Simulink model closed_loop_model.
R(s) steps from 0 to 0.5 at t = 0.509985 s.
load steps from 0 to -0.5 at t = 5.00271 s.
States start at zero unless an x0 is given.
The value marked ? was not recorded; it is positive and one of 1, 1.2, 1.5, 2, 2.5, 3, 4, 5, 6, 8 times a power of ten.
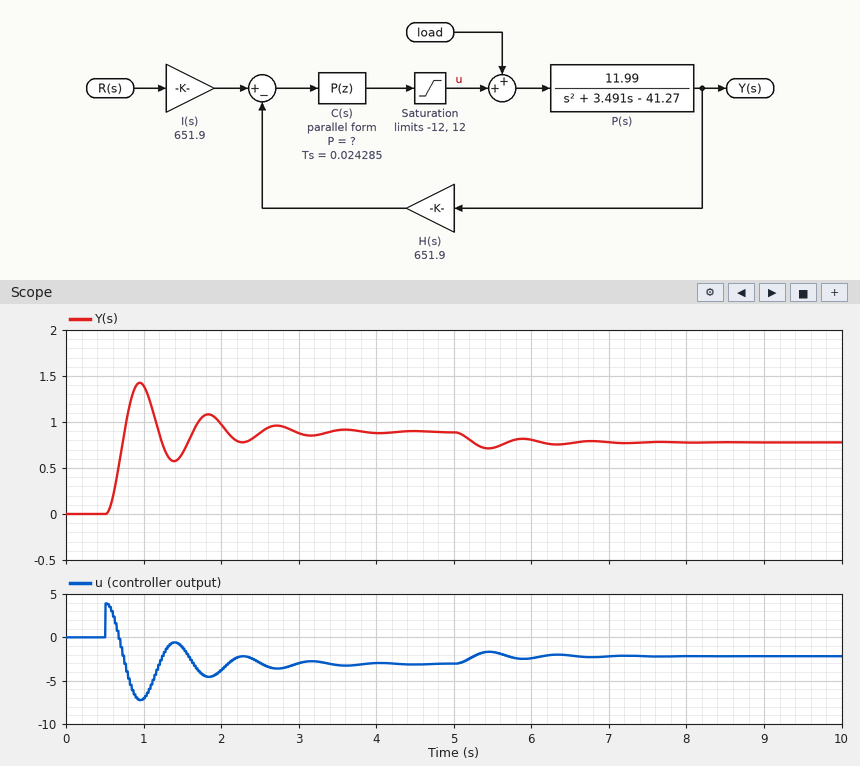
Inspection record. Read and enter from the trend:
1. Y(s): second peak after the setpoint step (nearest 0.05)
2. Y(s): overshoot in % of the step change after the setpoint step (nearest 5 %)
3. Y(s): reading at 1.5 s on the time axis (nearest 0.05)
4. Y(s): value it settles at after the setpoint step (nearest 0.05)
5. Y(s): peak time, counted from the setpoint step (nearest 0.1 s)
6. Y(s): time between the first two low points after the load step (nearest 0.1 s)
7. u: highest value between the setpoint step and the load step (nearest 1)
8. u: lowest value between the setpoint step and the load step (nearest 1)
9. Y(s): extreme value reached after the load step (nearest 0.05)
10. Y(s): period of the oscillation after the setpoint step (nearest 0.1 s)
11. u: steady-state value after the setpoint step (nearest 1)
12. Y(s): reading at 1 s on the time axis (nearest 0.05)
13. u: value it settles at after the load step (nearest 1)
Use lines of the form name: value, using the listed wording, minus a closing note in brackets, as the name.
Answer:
Y(s): second peak after the setpoint step: 1.10
Y(s): overshoot in % of the step change after the setpoint step: 60 %
Y(s): reading at 1.5 s on the time axis: 0.65
Y(s): value it settles at after the setpoint step: 0.90
Y(s): peak time, counted from the setpoint step: 0.4 s
Y(s): time between the first two low points after the load step: 0.9 s
u: highest value between the setpoint step and the load step: 4
u: lowest value between the setpoint step and the load step: -7
Y(s): extreme value reached after the load step: 0.70
Y(s): period of the oscillation after the setpoint step: 0.9 s
u: steady-state value after the setpoint step: -3
Y(s): reading at 1 s on the time axis: 1.40
u: value it settles at after the load step: -2
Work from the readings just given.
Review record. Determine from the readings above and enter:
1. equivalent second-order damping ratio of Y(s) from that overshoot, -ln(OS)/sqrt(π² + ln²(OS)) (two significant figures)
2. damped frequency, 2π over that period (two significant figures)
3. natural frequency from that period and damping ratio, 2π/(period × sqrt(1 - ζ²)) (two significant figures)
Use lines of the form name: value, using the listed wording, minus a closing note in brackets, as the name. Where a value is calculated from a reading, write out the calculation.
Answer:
equivalent second-order damping ratio of Y(s) from that overshoot, -ln(OS)/sqrt(π² + ln²(OS)): ln(0.6) = -0.511; 0.511 / sqrt(9.870 + 0.261) = 0.16
damped frequency, 2π over that period: 2π / 0.9 = 7.0 rad/s
natural frequency from that period and damping ratio, 2π/(period × sqrt(1 - ζ²)): 2π / (0.9 × sqrt(1 - 0.16²)) = 7.1 rad/s
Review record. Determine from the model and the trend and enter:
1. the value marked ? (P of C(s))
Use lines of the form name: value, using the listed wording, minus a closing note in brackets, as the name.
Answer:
the value marked ? (P of C(s)): 0.012
